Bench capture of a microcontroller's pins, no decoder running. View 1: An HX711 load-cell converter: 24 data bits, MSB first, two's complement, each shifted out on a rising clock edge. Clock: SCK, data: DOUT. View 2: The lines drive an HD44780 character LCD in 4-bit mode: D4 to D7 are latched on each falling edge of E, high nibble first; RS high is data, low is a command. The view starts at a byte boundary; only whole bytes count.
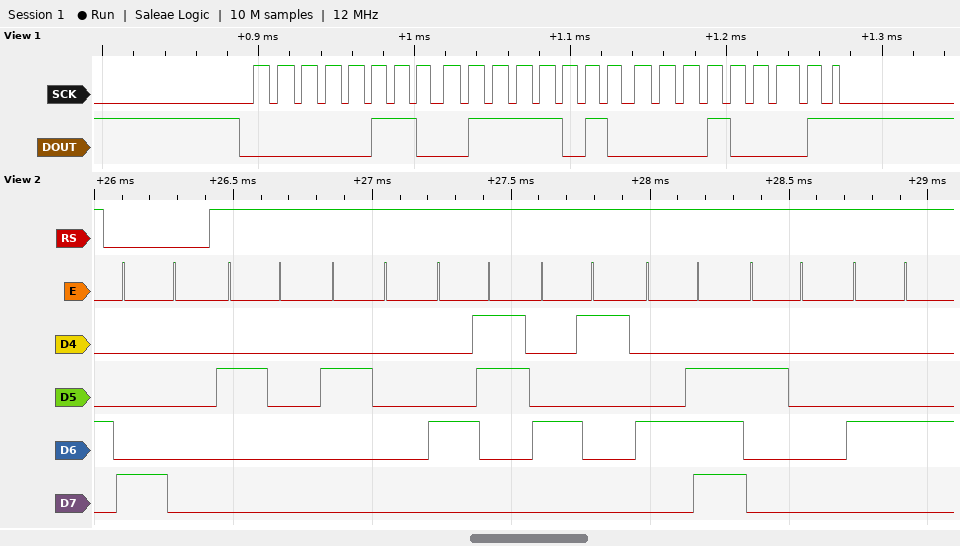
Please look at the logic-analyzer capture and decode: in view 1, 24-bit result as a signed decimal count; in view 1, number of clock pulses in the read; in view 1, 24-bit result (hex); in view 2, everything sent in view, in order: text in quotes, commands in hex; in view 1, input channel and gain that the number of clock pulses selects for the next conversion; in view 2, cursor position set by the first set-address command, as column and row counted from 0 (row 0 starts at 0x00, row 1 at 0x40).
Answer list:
424465
25
0x067A11
0x80 "  CAN D"
channel A, gain 128
column 0, row 0
